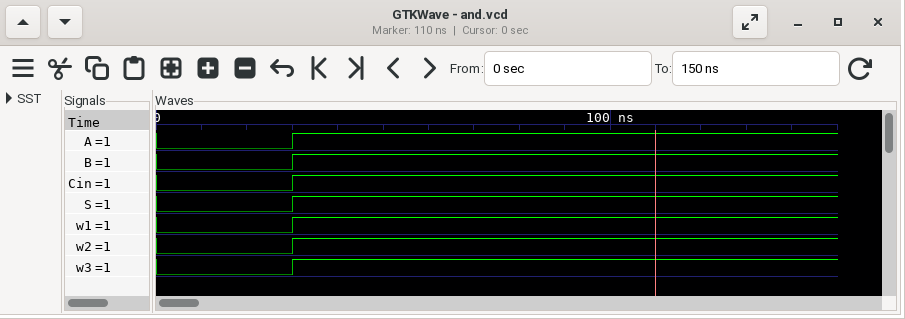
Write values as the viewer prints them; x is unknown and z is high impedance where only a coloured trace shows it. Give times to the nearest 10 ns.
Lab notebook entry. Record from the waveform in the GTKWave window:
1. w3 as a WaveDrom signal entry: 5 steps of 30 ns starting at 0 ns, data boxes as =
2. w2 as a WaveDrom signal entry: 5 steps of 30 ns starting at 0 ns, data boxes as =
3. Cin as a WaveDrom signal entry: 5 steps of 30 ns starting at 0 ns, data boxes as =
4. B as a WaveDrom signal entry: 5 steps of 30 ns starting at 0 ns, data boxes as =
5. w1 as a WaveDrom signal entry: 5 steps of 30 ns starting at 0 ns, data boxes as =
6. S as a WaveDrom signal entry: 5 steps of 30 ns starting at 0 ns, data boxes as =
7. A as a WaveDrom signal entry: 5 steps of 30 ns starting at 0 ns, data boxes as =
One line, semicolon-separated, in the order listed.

{name: 'w3', wave: '01...'}; {name: 'w2', wave: '01...'}; {name: 'Cin', wave: '01...'}; {name: 'B', wave: '01...'}; {name: 'w1', wave: '01...'}; {name: 'S', wave: '01...'}; {name: 'A', wave: '01...'}
